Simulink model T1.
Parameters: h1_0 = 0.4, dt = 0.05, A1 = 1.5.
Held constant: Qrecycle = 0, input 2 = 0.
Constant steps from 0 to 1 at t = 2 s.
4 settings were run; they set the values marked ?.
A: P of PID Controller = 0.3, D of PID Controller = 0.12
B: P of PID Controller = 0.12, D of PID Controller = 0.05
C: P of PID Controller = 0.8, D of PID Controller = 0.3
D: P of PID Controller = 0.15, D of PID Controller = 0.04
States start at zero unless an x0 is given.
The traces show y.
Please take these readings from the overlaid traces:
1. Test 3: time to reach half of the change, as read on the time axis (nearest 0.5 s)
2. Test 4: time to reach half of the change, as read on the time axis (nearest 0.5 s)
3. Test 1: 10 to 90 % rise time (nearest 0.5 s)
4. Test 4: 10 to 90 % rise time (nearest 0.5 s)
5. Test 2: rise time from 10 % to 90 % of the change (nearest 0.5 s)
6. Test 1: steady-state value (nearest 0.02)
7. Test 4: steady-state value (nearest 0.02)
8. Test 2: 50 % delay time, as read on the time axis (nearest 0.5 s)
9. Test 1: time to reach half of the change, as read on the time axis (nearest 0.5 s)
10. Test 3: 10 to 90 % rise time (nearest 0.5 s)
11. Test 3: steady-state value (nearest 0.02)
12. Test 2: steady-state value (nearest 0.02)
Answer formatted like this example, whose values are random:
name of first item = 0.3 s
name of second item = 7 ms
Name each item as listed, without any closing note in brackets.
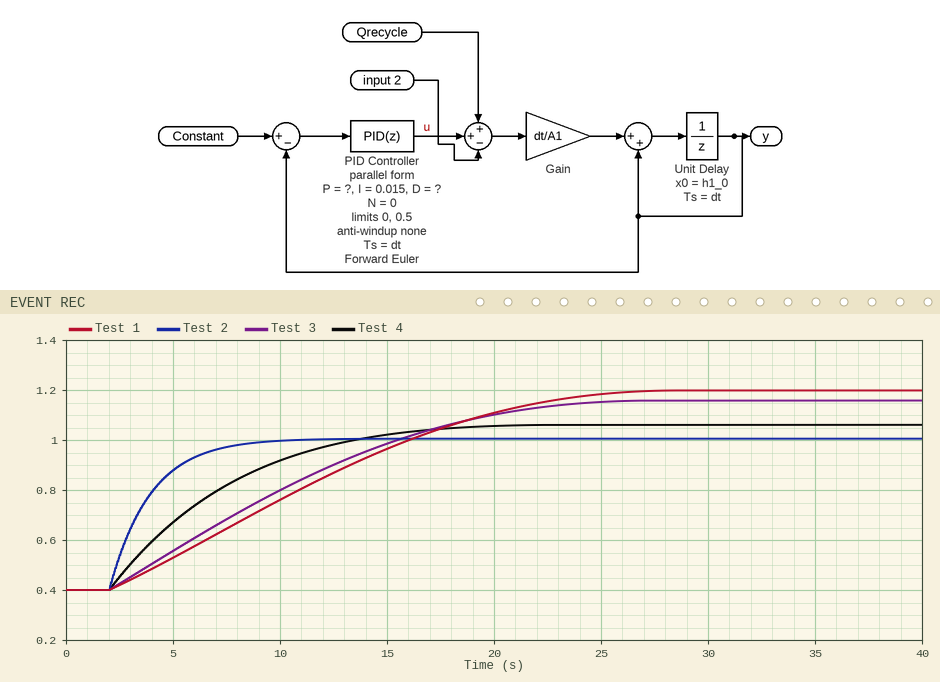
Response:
Test 3: time to reach half of the change, as read on the time axis = 9.5 s
Test 4: time to reach half of the change, as read on the time axis = 6.0 s
Test 1: 10 to 90 % rise time = 16.5 s
Test 4: 10 to 90 % rise time = 10.5 s
Test 2: rise time from 10 % to 90 % of the change = 4.0 s
Test 1: steady-state value = 1.20
Test 4: steady-state value = 1.06
Test 2: 50 % delay time, as read on the time axis = 3.5 s
Test 1: time to reach half of the change, as read on the time axis = 11.0 s
Test 3: 10 to 90 % rise time = 15.5 s
Test 3: steady-state value = 1.16
Test 2: steady-state value = 1.00
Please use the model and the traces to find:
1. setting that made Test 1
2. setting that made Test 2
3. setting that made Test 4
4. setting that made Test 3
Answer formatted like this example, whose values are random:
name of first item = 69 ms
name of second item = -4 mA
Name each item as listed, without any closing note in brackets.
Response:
setting that made Test 1 = B
setting that made Test 2 = C
setting that made Test 4 = A
setting that made Test 3 = D
